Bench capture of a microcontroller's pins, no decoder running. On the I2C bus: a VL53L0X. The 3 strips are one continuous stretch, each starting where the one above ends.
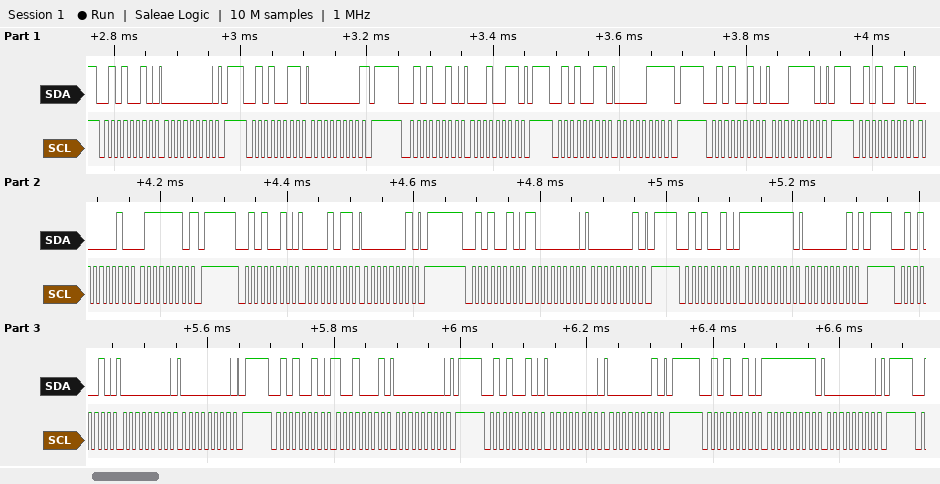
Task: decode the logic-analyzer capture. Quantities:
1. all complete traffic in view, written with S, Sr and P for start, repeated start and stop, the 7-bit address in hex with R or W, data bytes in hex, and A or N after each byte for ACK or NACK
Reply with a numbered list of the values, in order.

1. S 29W A 00 A P S 29R A 00 N P S 29W A 13 A P S 29R A 07 N P S 29W A 1E A P S 29R A 02 A 7E N P S 29W A 0B A 01 A P S 29W A 80 A 01 A P S 29W A FF A 01 A P S 29W A 00 A 00 A P S 29W A 91 A 00 A P S 29W A 00 A 01 A P S 29W A FF A 00 A P
